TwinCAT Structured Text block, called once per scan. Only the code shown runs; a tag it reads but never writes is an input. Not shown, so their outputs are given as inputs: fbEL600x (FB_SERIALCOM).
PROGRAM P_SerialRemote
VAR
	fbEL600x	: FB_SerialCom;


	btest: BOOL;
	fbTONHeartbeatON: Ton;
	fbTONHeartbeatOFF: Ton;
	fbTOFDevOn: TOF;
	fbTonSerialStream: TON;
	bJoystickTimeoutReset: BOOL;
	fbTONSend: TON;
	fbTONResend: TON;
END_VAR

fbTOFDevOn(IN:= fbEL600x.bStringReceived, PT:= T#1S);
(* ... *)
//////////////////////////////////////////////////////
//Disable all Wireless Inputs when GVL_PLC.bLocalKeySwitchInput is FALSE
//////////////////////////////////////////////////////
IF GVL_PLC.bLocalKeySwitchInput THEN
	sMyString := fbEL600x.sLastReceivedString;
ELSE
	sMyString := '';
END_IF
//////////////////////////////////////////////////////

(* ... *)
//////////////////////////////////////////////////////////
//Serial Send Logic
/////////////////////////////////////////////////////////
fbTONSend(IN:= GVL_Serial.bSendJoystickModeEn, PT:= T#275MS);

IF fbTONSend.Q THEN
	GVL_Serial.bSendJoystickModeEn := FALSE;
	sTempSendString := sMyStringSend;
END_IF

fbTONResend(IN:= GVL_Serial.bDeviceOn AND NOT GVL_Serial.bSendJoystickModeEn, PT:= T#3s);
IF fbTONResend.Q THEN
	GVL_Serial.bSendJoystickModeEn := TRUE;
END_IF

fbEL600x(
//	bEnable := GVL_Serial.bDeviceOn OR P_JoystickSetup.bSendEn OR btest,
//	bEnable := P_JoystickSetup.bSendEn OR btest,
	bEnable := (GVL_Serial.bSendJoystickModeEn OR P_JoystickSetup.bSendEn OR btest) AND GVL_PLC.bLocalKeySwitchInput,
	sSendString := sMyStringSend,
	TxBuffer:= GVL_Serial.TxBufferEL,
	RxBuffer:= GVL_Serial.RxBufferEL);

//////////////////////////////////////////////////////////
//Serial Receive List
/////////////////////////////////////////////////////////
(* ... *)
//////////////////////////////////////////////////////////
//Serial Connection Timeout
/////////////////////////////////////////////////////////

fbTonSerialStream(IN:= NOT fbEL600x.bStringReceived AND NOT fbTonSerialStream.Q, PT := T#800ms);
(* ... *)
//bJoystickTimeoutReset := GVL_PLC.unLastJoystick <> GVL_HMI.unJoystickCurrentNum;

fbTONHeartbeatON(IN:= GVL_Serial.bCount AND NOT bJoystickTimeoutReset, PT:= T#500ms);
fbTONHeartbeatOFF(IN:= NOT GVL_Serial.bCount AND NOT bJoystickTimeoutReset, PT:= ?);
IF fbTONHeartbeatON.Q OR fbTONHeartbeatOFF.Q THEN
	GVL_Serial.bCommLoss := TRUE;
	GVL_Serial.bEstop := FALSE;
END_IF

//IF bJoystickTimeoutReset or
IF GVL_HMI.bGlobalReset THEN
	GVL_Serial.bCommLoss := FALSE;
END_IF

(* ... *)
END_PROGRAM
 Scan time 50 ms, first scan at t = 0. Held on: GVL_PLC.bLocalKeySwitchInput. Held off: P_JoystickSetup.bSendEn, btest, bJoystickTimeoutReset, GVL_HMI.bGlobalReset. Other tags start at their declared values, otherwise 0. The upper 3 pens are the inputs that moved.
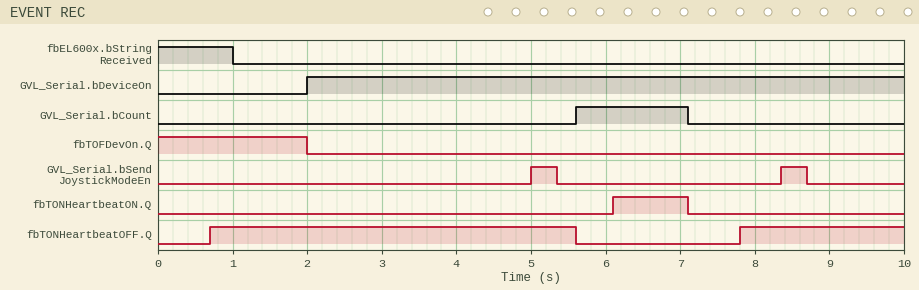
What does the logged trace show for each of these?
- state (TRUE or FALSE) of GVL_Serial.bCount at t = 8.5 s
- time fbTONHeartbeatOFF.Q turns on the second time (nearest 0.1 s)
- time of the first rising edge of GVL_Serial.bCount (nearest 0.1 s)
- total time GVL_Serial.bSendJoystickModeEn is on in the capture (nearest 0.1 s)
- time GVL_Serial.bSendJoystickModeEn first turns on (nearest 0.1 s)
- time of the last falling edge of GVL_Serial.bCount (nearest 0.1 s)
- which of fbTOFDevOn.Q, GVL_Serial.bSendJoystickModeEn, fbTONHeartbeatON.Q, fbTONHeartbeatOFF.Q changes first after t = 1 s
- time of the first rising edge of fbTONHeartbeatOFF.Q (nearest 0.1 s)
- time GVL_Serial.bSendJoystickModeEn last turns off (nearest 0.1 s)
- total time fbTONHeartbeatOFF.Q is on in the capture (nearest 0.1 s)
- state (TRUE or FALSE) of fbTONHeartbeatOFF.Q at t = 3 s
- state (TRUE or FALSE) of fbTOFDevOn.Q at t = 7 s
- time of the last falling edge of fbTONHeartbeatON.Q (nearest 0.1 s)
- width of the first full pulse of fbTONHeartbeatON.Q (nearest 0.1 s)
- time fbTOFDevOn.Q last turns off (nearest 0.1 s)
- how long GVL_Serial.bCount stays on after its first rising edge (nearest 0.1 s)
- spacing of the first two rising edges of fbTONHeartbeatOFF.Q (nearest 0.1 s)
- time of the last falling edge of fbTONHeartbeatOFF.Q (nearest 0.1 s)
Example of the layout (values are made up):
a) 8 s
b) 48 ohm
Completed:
a) FALSE
b) 7.8 s
c) 5.6 s
d) 0.7 s
e) 5.0 s
f) 7.1 s
g) fbTOFDevOn.Q
h) 0.7 s
i) 8.7 s
j) 7.1 s
k) TRUE
l) FALSE
m) 7.1 s
n) 1.0 s
o) 2.0 s
p) 1.5 s
q) 7.1 s
r) 5.6 s
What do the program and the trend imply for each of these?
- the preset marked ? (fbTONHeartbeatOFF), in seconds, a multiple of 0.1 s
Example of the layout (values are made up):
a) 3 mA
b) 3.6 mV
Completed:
a) 0.7 s
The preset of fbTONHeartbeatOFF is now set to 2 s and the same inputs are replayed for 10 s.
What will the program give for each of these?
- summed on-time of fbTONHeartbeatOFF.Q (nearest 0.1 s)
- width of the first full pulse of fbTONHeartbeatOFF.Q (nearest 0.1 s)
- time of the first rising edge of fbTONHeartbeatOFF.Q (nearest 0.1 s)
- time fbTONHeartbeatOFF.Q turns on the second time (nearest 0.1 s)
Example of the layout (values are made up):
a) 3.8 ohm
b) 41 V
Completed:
a) 4.5 s
b) 3.6 s
c) 2.0 s
d) 9.1 s
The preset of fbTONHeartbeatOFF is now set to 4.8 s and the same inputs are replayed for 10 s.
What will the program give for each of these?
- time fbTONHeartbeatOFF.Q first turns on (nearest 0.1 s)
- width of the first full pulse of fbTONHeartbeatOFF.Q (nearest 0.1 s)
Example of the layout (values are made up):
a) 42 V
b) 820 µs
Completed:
a) 4.8 s
b) 0.8 s
